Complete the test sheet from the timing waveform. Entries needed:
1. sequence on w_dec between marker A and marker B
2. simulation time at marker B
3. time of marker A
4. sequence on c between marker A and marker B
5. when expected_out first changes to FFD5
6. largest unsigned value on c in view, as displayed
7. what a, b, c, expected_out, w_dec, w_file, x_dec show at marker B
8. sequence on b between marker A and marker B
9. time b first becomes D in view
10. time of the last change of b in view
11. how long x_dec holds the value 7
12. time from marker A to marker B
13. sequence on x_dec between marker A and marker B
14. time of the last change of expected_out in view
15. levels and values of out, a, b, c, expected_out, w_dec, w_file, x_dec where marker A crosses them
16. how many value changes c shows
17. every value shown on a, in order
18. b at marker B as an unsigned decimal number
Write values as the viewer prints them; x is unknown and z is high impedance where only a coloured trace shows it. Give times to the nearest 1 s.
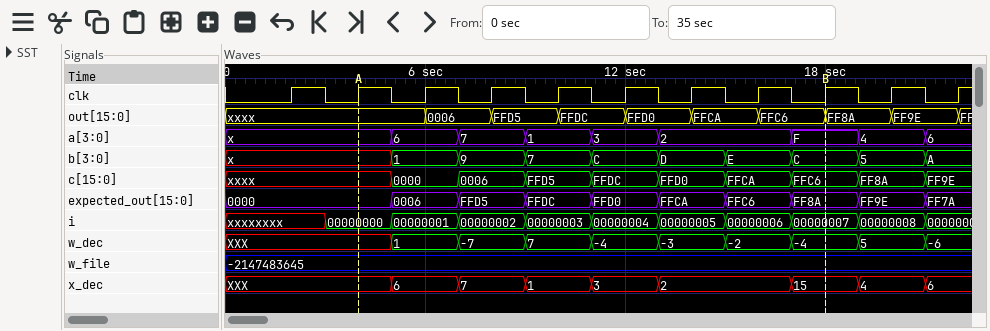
XXX, 1, -7, 7, -4, -3, -2, -4
18 s
4 s
xxxx, 0000, 0006, FFD5, FFDC, FFD0, FFCA, FFC6
7 s
FFDC
a=F, b=C, c=FFC6, expected_out=FF8A, w_dec=-4, w_file=-2147483645, x_dec=15
x, 1, 9, 7, C, D, E, C
13 s
21 s
2 s
14 s
XXX, 6, 7, 1, 3, 2, 15
21 s
out=xxxx, a=x, b=x, c=xxxx, expected_out=0000, w_dec=XXX, w_file=-2147483645, x_dec=XXX
9
x, 6, 7, 1, 3, 2, F, 4, 6
12
